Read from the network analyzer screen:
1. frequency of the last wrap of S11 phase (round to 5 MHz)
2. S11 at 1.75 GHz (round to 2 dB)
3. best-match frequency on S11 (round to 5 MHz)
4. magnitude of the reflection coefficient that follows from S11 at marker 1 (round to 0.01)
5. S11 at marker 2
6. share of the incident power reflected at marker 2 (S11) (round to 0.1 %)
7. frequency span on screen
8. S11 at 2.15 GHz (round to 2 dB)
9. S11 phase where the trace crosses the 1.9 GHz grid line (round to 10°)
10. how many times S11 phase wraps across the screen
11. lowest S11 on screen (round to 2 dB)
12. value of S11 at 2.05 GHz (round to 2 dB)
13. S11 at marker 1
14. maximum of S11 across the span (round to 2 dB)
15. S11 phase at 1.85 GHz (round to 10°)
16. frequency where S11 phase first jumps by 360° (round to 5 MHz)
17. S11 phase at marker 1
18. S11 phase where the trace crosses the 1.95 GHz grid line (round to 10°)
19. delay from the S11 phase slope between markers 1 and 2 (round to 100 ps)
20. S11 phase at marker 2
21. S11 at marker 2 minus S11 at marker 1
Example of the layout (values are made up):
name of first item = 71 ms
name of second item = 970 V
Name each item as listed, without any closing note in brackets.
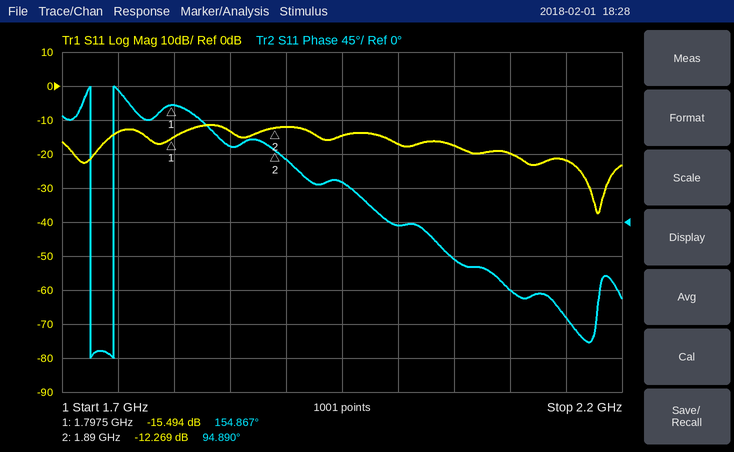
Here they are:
frequency of the last wrap of S11 phase = 1.745 GHz
S11 at 1.75 GHz = -14 dB
best-match frequency on S11 = 2.180 GHz
magnitude of the reflection coefficient that follows from S11 at marker 1 = 0.17
S11 at marker 2 = -12.269 dB
share of the incident power reflected at marker 2 (S11) = 5.9 %
frequency span on screen = 500 MHz
S11 at 2.15 GHz = -22 dB
S11 phase where the trace crosses the 1.9 GHz grid line = 80°
how many times S11 phase wraps across the screen = 2
lowest S11 on screen = -38 dB
value of S11 at 2.05 GHz = -18 dB
S11 at marker 1 = -15.494 dB
maximum of S11 across the span = -12 dB
S11 phase at 1.85 GHz = 100°
frequency where S11 phase first jumps by 360° = 1.725 GHz
S11 phase at marker 1 = 154.867°
S11 phase where the trace crosses the 1.95 GHz grid line = 50°
delay from the S11 phase slope between markers 1 and 2 = 1.8 ns
S11 phase at marker 2 = 94.890°
S11 at marker 2 minus S11 at marker 1 = 3.225 dB
